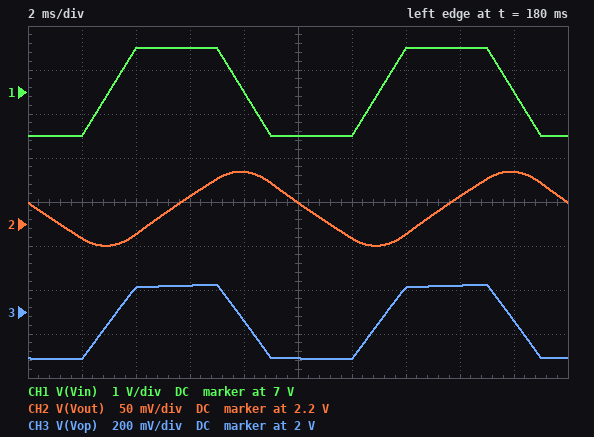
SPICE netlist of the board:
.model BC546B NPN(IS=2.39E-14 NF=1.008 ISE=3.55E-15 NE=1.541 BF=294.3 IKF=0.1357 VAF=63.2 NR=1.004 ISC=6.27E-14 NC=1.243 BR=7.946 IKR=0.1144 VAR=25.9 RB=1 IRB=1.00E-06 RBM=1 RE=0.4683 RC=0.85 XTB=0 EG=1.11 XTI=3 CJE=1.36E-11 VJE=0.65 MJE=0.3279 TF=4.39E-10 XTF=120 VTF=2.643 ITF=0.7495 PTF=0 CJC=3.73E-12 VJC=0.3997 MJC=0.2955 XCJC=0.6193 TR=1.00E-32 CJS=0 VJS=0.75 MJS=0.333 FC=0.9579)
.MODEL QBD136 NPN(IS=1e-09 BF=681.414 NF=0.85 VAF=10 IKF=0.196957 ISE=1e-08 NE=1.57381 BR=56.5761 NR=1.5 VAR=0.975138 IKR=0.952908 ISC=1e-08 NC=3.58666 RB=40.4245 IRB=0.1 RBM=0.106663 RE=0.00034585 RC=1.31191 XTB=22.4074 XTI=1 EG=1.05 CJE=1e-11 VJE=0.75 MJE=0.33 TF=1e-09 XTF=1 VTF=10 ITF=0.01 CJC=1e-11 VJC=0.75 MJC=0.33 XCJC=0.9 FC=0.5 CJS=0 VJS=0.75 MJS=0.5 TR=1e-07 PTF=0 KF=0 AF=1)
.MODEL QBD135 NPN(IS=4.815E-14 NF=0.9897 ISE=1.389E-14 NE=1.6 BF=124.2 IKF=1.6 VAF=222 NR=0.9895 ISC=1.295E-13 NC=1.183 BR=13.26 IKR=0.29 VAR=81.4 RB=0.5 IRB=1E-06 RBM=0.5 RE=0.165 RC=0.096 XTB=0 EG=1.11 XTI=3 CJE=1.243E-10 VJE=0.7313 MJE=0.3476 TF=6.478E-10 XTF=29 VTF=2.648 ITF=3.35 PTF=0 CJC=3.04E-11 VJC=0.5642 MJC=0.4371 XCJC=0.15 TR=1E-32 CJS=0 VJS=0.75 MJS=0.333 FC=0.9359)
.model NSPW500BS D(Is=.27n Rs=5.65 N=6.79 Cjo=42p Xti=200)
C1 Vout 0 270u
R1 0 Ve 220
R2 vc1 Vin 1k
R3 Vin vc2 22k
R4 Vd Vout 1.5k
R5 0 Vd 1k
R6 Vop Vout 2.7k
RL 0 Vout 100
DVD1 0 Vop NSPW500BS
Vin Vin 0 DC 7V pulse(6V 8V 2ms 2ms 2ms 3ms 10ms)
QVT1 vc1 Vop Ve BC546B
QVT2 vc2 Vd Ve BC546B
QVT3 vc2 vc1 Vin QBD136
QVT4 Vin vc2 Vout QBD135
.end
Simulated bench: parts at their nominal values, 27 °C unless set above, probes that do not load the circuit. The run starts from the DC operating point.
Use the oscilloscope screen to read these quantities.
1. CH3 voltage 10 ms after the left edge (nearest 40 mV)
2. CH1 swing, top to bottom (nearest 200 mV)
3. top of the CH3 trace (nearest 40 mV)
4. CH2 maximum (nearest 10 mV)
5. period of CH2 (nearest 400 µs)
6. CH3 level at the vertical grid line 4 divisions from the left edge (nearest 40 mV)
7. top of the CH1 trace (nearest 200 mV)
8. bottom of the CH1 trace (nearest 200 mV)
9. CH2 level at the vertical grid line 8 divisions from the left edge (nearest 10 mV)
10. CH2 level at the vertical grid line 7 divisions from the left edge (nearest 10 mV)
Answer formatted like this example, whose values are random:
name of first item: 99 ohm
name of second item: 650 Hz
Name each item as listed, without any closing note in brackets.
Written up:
CH3 voltage 10 ms after the left edge: 1.80 V
CH1 swing, top to bottom: 2.0 V
top of the CH3 trace: 2.12 V
CH2 maximum: 2.26 V
period of CH2: 10.0 ms
CH3 level at the vertical grid line 4 divisions from the left edge: 1.96 V
top of the CH1 trace: 8.0 V
bottom of the CH1 trace: 6.0 V
CH2 level at the vertical grid line 8 divisions from the left edge: 2.23 V
CH2 level at the vertical grid line 7 divisions from the left edge: 2.19 V
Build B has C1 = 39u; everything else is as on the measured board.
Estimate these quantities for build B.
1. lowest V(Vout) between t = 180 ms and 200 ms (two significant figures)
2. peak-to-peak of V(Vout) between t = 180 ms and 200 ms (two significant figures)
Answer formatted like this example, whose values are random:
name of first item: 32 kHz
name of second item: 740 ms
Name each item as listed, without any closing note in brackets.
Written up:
lowest V(Vout) between t = 180 ms and 200 ms: 2.0 V
peak-to-peak of V(Vout) between t = 180 ms and 200 ms: 470 mV
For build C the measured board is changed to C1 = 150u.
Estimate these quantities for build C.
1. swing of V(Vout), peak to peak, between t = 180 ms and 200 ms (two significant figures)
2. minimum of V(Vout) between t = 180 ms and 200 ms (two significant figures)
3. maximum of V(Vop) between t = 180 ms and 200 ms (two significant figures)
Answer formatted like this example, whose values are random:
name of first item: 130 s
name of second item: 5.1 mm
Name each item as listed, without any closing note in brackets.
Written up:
swing of V(Vout), peak to peak, between t = 180 ms and 200 ms: 150 mV
minimum of V(Vout) between t = 180 ms and 200 ms: 2.1 V
maximum of V(Vop) between t = 180 ms and 200 ms: 2.1 V
